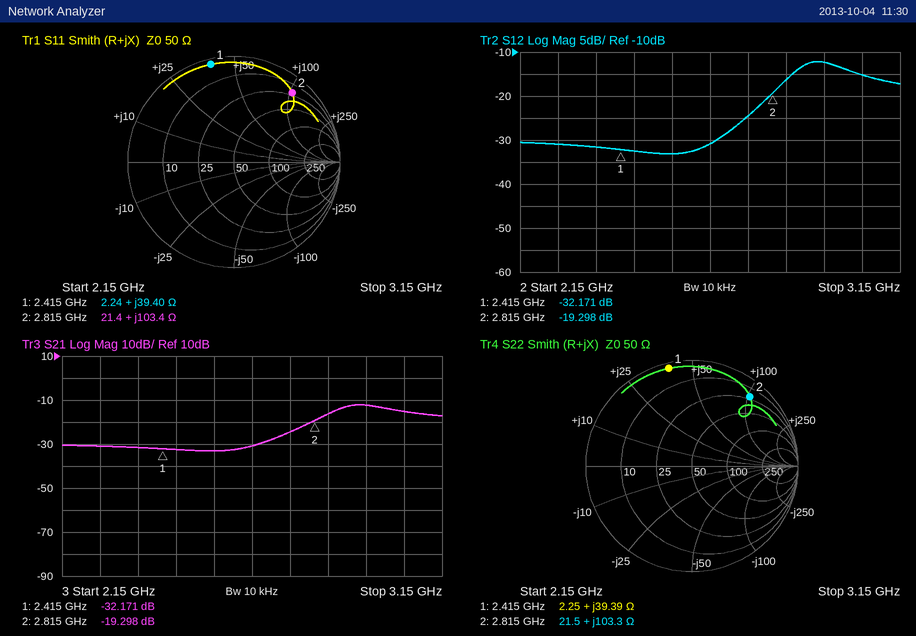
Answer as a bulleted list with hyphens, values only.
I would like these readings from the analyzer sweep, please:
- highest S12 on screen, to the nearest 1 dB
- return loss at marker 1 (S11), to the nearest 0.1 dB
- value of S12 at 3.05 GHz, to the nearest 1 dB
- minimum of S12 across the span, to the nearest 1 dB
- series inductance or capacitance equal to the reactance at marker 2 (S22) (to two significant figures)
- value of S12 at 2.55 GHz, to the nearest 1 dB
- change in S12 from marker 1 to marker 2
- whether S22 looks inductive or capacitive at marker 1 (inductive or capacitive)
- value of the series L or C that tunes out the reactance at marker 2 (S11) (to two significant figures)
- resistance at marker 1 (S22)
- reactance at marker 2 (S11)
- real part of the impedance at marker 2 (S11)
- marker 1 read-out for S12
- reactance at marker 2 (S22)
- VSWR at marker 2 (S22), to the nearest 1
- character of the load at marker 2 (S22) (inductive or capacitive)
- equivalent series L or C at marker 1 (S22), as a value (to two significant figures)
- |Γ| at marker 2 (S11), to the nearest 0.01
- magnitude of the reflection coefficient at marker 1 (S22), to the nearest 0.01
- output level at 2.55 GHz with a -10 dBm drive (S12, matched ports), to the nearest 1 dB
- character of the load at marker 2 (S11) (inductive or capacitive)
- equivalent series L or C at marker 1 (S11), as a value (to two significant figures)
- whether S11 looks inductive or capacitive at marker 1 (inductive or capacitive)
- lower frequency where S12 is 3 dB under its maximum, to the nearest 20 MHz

- -12 dB
- 0.5 dB
- -15 dB
- -33 dB
- 5.8 nH
- -33 dB
- 12.873 dB
- inductive
- 550 fF
- 2.25 Ω
- +103.4 Ω
- 21.4 Ω
- -32.171 dB
- +103.3 Ω
- 13
- inductive
- 2.6 nH
- 0.85
- 0.95
- -43 dBm
- inductive
- 2.6 nH
- inductive
- 2.86 GHz
